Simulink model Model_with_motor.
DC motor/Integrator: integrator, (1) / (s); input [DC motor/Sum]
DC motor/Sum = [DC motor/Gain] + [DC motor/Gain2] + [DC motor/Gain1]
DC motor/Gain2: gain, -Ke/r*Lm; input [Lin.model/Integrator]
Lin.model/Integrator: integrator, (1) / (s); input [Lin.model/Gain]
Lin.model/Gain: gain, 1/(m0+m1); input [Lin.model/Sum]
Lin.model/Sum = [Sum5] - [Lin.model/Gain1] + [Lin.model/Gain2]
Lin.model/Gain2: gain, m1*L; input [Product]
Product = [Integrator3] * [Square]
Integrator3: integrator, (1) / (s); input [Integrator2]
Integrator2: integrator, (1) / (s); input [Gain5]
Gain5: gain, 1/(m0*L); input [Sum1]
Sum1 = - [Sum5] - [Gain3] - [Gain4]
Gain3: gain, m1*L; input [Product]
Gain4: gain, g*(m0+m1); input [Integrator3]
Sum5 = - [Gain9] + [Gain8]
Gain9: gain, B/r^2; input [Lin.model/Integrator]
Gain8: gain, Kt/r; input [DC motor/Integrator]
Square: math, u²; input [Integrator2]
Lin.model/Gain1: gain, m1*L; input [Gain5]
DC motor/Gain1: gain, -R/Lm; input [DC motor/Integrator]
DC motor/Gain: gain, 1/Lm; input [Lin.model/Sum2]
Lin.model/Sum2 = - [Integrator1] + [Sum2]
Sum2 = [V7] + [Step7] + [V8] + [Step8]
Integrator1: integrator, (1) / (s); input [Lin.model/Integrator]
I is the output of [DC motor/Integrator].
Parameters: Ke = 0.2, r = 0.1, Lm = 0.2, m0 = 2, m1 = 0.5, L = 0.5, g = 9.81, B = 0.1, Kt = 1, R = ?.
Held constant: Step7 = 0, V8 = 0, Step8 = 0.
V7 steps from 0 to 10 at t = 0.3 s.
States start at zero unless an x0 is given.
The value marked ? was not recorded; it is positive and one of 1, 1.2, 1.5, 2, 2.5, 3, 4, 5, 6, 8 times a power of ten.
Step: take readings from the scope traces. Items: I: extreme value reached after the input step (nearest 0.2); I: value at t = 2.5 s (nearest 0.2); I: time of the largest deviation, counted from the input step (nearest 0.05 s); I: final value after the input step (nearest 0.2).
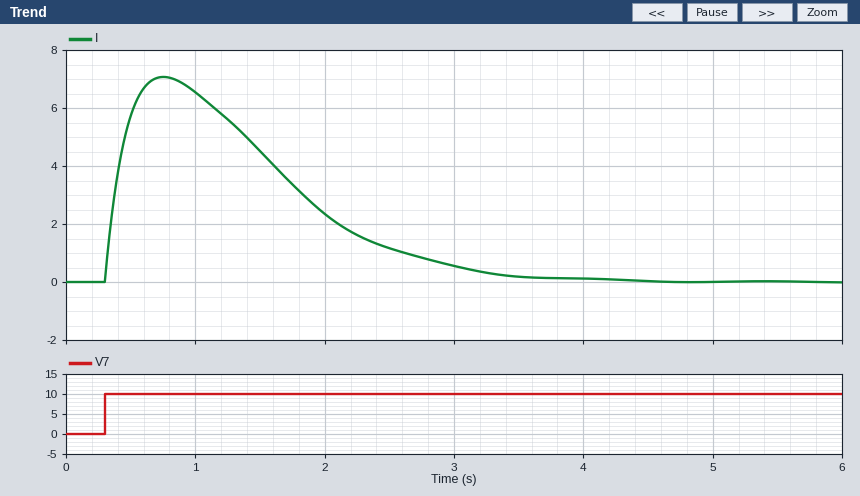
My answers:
7.0
1.2
0.45 s
0.0
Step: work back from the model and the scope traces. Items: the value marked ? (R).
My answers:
1.2
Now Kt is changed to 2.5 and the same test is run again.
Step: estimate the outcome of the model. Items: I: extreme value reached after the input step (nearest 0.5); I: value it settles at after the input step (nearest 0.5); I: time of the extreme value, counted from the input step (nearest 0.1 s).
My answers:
6.5
0.0
0.4 s
